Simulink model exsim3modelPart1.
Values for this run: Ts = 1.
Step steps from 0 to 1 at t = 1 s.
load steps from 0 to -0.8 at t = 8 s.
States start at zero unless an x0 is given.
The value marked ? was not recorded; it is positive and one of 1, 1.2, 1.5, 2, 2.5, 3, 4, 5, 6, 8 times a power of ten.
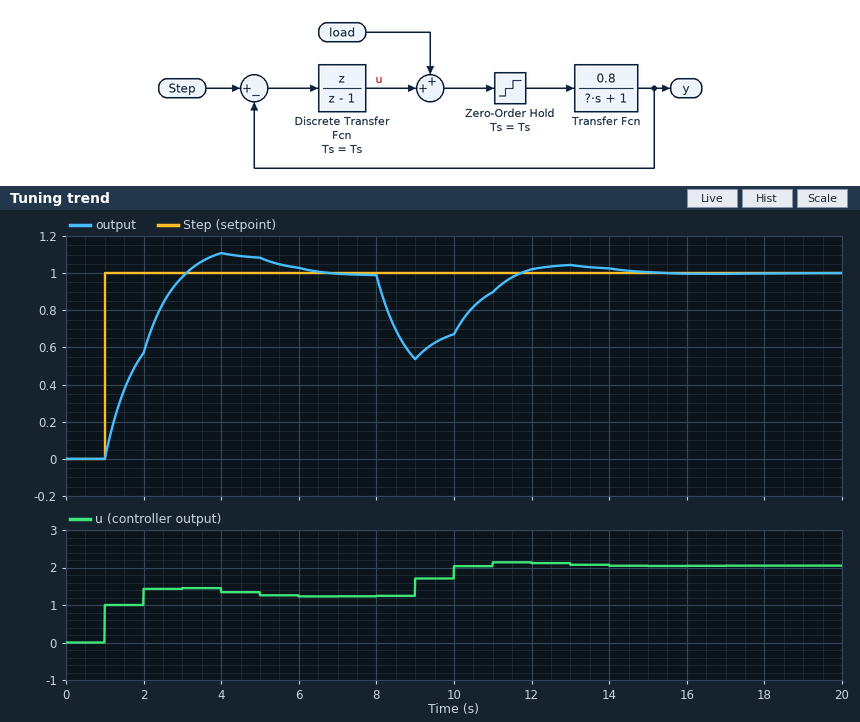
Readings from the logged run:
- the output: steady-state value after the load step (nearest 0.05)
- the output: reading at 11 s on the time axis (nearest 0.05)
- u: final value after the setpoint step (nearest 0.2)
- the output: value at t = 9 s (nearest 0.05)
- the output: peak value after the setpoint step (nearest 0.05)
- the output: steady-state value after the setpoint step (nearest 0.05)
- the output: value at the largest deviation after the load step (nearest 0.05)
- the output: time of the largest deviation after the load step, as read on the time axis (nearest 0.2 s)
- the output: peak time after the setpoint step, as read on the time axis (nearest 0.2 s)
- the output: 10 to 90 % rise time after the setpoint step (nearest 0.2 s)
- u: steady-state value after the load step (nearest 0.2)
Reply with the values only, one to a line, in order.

1.00
0.90
1.2
0.55
1.10
1.00
0.55
9.0 s
4.0 s
1.6 s
2.0
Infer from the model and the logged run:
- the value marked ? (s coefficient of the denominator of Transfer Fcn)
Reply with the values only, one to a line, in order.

0.8
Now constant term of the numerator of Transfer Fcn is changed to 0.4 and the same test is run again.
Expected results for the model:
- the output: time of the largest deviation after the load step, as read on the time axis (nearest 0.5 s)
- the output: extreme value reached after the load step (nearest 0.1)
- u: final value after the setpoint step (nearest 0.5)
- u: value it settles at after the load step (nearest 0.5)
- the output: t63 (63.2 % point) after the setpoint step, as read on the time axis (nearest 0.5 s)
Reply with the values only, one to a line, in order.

10.0 s
0.8
2.5
3.5
3.0 s
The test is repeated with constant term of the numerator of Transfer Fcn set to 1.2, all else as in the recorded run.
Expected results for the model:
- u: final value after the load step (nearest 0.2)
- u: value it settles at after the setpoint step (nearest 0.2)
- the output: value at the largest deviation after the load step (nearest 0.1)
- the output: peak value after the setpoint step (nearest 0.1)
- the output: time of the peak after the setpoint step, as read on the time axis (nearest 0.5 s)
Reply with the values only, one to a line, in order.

1.6
0.8
0.3
1.2
3.0 s
